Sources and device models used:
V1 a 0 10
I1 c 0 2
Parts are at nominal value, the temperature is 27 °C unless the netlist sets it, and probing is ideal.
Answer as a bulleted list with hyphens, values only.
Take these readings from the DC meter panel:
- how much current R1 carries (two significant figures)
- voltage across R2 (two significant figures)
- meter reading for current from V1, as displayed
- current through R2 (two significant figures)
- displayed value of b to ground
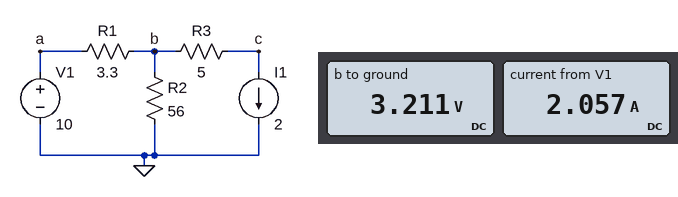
- 2.1 A
- 3.2 V
- 2.057 A
- 57 mA
- 3.211 V
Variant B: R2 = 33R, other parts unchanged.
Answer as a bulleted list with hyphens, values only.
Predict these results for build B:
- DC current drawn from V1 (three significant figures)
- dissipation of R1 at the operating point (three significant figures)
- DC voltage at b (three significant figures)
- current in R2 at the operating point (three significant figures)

- 2.09 A
- 14.5 W
- 3.09 V
- 93.7 mA
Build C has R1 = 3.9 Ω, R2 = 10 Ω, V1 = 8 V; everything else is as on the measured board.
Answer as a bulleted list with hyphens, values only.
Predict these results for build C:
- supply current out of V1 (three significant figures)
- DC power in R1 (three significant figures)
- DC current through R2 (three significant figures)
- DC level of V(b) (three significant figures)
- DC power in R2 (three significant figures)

- 2.01 A
- 15.8 W
- 14.4 mA
- 144 mV
- 2.07 mW
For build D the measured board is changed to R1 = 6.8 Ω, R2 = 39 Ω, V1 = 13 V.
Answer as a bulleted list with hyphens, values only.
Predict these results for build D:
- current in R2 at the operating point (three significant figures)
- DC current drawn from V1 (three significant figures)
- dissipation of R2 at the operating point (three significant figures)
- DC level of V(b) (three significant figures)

- 13.1 mA
- 1.99 A
- 6.69 mW
- -511 mV
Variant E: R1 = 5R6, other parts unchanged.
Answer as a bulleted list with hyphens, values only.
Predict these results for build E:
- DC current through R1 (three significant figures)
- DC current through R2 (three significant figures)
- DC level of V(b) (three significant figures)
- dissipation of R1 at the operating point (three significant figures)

- 1.98 A
- 19.5 mA
- -1.09 V
- 22.0 W
